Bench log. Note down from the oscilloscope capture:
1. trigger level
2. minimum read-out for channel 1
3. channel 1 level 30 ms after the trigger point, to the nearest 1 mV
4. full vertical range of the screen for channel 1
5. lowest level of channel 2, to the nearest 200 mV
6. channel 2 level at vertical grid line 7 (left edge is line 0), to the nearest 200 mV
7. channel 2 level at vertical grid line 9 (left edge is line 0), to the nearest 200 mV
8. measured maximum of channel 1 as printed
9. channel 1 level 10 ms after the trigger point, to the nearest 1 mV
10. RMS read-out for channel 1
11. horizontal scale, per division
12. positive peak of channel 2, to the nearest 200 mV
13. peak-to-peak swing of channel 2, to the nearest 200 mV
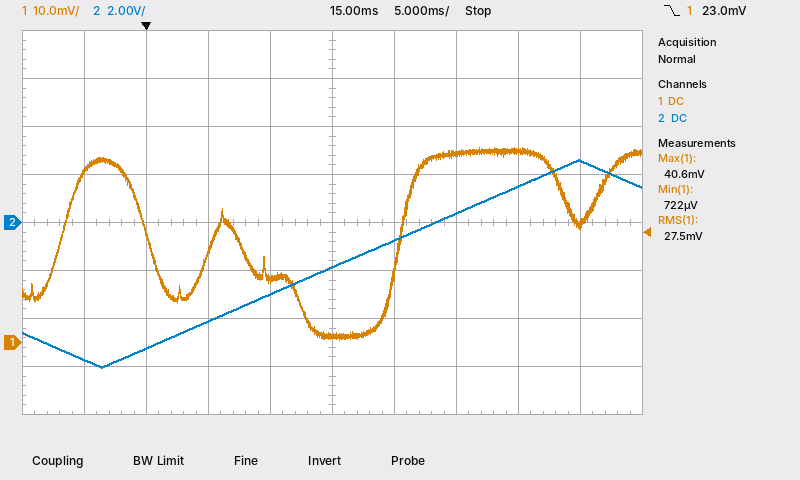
23.0 mV
722 µV
40 mV
80 mV
-6.0 V
400 mV
2.6 V
40.6 mV
13 mV
27.5 mV
5 ms
2.6 V
8.6 V
